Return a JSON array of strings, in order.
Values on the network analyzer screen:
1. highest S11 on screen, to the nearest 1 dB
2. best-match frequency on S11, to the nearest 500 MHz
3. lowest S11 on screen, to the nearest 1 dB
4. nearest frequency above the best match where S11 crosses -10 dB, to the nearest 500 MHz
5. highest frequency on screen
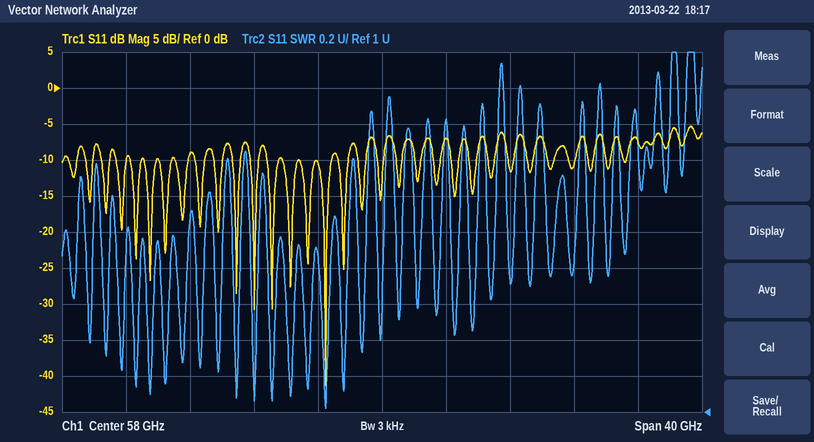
["-5 dB", "54.5 GHz", "-41 dB", "55.0 GHz", "78 GHz"]
